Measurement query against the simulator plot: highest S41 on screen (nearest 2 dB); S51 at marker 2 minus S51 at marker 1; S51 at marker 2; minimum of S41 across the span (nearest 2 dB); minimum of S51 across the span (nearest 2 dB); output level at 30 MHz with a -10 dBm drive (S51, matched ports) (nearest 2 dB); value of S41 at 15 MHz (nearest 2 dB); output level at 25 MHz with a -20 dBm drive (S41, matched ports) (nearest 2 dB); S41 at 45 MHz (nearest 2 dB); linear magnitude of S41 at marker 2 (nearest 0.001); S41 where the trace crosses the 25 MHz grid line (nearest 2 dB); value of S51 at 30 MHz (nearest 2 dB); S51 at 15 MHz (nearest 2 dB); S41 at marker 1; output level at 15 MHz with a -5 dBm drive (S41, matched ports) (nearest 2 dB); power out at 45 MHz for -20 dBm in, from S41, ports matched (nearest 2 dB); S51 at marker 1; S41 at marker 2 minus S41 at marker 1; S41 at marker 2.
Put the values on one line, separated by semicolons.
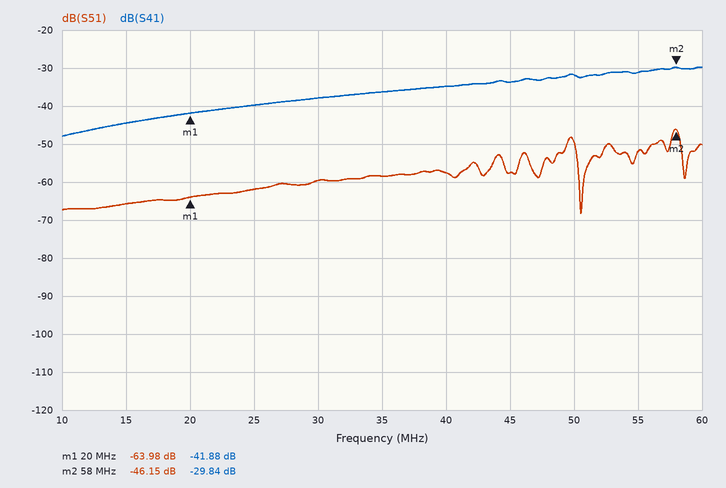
-30 dB; 17.83 dB; -46.15 dB; -48 dB; -68 dB; -70 dBm; -44 dB; -60 dBm; -34 dB; 0.032; -40 dB; -60 dB; -66 dB; -41.88 dB; -50 dBm; -54 dBm; -63.98 dB; 12.04 dB; -29.84 dB
